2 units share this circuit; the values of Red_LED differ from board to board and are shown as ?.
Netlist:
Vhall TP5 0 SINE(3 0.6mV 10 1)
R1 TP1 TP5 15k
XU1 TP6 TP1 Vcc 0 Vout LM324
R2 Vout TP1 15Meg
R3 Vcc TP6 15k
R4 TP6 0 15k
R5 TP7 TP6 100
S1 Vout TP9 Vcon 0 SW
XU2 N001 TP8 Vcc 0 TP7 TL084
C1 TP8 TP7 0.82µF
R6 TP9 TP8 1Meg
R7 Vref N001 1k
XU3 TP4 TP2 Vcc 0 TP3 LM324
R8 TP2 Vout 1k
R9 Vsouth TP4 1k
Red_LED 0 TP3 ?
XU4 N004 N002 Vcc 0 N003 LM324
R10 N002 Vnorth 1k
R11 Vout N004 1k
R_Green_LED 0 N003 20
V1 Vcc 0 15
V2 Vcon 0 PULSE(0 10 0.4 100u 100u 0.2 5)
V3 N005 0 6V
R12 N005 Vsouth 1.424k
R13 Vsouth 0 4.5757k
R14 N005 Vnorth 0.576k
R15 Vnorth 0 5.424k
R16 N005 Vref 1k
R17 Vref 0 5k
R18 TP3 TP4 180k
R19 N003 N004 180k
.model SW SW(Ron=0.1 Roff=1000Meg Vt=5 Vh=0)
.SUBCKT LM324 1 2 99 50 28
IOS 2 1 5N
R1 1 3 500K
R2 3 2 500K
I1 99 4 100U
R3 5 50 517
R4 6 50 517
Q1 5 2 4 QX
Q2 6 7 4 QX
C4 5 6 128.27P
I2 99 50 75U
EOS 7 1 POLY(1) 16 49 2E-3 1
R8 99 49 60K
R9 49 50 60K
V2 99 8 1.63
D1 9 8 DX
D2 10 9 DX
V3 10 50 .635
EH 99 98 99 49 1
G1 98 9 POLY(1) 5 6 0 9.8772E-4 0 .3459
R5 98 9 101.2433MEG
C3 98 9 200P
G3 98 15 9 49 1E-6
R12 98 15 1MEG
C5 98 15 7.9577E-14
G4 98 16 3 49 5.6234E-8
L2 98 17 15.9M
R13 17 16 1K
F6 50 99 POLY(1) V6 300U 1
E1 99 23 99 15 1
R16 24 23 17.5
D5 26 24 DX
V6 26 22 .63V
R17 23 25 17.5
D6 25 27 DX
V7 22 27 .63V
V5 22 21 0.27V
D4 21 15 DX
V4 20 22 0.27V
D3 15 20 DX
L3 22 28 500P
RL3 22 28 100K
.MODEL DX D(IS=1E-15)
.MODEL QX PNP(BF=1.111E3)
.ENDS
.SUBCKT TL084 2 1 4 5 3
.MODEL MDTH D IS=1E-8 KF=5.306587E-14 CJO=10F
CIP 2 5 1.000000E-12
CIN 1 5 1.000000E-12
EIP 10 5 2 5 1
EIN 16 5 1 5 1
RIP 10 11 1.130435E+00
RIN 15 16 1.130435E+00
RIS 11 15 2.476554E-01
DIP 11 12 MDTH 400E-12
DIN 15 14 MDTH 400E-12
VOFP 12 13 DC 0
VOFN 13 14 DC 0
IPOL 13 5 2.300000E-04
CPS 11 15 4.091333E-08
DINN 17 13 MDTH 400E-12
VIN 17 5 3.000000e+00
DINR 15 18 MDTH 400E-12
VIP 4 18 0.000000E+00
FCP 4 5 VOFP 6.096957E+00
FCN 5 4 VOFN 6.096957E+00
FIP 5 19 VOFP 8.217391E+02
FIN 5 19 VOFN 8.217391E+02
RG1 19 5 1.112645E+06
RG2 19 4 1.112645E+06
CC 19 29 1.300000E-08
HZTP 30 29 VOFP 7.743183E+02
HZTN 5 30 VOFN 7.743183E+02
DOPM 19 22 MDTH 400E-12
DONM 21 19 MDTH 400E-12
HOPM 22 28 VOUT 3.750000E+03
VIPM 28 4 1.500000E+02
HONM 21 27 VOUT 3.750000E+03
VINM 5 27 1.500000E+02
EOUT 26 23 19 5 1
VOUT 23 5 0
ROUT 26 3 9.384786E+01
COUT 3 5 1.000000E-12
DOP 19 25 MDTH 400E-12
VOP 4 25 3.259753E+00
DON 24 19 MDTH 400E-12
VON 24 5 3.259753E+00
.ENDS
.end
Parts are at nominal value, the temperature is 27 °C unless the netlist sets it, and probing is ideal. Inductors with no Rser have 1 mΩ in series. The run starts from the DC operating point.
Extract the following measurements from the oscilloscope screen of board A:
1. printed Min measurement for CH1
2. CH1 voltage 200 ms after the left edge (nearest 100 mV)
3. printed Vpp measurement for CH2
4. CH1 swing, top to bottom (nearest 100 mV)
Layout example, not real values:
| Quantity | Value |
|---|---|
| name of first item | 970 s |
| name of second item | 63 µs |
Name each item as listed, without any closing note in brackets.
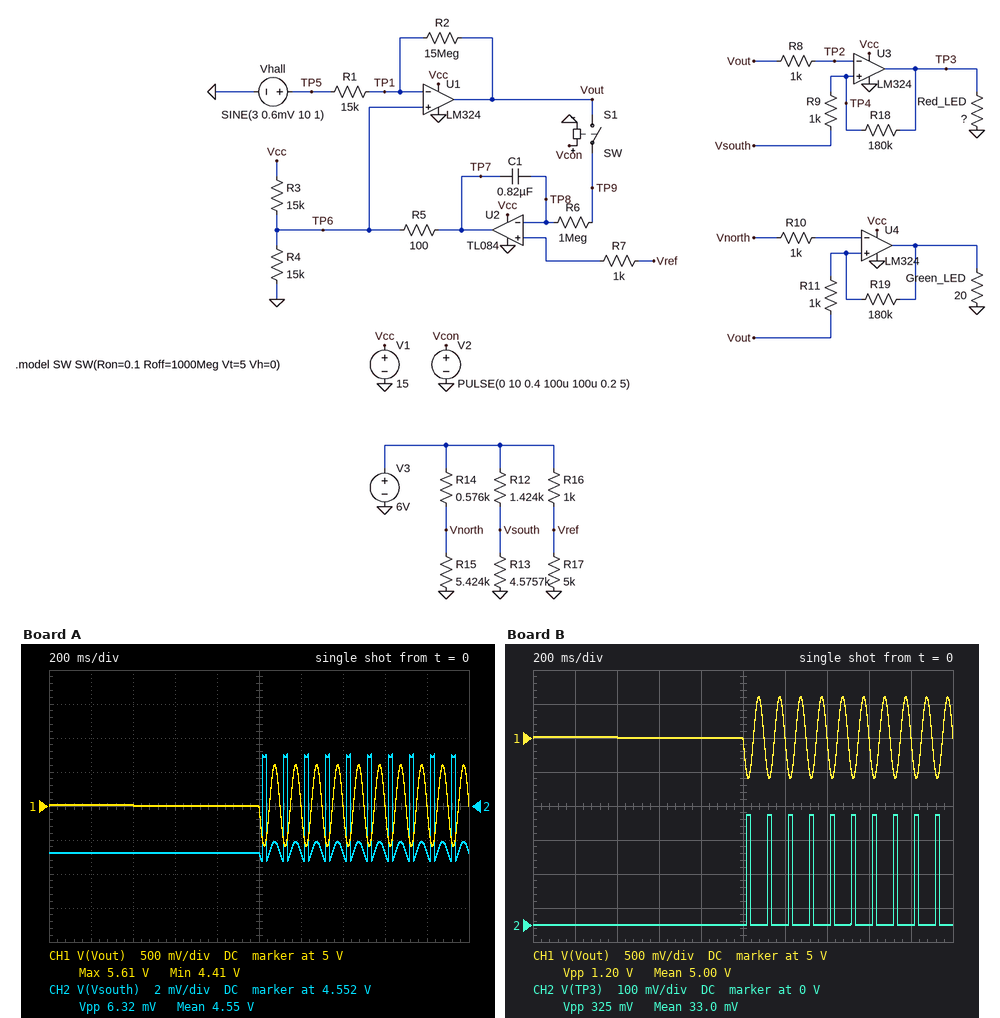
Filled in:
| Quantity | Value |
|---|---|
| printed Min measurement for CH1 | 4.41 V |
| CH1 voltage 200 ms after the left edge | 5.0 V |
| printed Vpp measurement for CH2 | 6.32 mV |
| CH1 swing, top to bottom | 1.2 V |
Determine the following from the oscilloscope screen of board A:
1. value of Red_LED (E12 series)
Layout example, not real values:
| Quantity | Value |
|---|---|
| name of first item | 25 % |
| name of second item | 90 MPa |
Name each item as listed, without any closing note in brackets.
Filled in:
| Quantity | Value |
|---|---|
| value of Red_LED | 27 Ω |
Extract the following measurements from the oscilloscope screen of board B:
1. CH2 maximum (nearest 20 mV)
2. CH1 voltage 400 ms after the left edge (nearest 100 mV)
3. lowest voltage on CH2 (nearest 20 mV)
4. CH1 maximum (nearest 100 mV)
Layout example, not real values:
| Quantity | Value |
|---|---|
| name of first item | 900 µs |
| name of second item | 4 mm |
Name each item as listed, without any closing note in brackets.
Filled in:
| Quantity | Value |
|---|---|
| CH2 maximum | 320 mV |
| CH1 voltage 400 ms after the left edge | 5.0 V |
| lowest voltage on CH2 | 0 V |
| CH1 maximum | 5.6 V |
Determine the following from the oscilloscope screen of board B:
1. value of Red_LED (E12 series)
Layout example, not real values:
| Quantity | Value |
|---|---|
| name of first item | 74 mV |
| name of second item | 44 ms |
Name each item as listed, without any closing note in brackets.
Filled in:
| Quantity | Value |
|---|---|
| value of Red_LED | 8.2 Ω |
